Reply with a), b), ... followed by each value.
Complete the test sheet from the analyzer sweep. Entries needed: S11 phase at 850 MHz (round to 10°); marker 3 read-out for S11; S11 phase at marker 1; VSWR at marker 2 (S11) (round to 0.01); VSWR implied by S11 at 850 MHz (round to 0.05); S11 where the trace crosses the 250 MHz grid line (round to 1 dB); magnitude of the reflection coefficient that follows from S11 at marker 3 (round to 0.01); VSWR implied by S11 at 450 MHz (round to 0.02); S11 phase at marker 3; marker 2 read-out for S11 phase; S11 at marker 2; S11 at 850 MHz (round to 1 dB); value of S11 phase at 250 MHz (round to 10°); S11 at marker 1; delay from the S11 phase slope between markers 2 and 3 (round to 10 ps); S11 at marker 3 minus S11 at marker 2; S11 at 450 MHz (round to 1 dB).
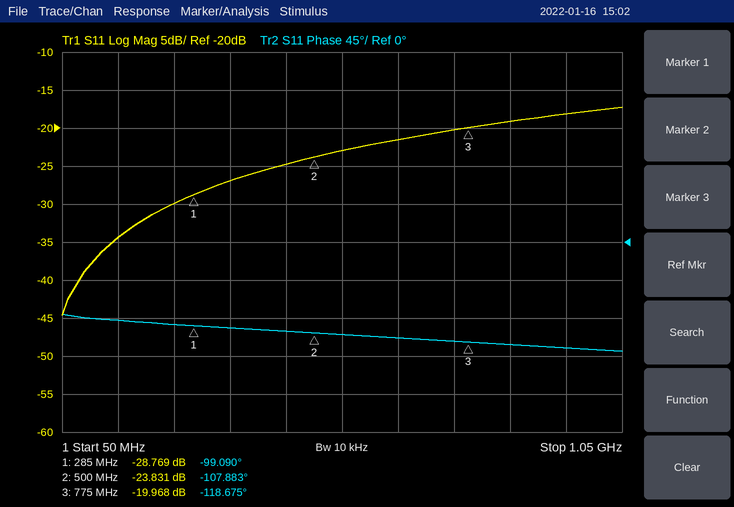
a) -120°
b) -19.968 dB
c) -99.090°
d) 1.14
e) 1.25
f) -30 dB
g) 0.10
h) 1.12
i) -118.675°
j) -107.883°
k) -23.831 dB
l) -19 dB
m) -100°
n) -28.769 dB
o) 110 ps
p) 3.863 dB
q) -25 dB
